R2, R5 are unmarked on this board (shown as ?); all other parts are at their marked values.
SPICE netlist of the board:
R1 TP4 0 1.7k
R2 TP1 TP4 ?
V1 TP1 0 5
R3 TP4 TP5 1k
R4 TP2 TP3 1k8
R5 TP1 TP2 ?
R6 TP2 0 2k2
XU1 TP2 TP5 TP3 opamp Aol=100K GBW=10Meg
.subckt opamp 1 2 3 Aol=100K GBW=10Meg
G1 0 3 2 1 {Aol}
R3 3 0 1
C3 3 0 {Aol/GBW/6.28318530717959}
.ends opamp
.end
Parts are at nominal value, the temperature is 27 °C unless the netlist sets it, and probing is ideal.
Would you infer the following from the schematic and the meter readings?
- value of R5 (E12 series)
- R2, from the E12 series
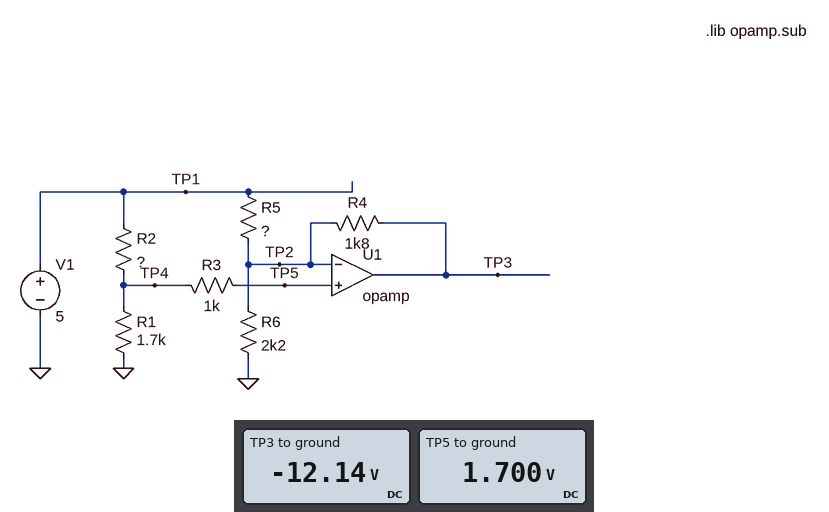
390 Ω
3.3 kΩ
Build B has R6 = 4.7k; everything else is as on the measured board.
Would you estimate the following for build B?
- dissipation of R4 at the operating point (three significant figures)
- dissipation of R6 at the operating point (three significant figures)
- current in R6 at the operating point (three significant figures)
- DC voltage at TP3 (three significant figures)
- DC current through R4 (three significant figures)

118 mW
615 µW
362 µA
-12.9 V
8.10 mA
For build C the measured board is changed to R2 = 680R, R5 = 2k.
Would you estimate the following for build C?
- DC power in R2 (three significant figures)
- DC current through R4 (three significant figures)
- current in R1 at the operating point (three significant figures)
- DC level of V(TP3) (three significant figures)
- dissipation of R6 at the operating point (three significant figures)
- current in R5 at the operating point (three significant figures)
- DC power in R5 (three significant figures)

3.00 mW
909 µA
2.10 mA
5.21 V
5.80 mW
714 µA
1.02 mW
